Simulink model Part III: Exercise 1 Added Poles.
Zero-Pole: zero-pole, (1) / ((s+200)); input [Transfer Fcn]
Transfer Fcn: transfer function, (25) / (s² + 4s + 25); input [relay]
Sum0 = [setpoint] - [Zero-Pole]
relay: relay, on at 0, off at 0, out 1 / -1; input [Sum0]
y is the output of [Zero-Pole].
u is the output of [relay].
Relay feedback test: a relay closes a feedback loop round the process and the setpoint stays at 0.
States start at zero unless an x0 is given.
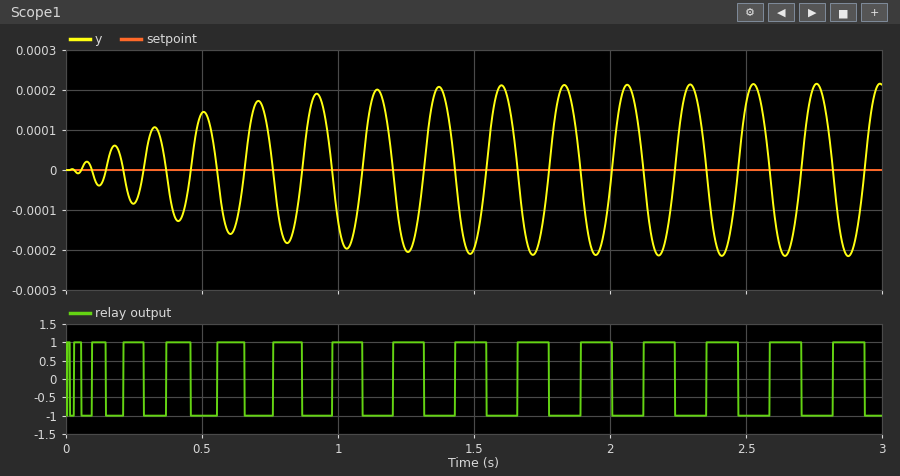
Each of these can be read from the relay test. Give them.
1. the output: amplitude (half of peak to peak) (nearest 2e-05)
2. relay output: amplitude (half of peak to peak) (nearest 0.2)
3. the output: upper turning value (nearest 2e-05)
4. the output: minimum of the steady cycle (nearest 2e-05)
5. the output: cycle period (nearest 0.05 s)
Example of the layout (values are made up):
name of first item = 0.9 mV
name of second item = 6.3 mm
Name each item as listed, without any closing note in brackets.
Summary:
the output: amplitude (half of peak to peak) = 0.00022
relay output: amplitude (half of peak to peak) = 1.0
the output: upper turning value = 0.00022
the output: minimum of the steady cycle = -0.00022
the output: cycle period = 0.25 s
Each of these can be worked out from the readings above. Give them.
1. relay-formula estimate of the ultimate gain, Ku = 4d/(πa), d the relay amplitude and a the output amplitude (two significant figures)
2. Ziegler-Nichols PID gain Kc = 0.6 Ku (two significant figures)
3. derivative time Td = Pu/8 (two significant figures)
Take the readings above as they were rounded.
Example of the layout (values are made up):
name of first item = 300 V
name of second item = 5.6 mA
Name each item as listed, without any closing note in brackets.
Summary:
relay-formula estimate of the ultimate gain, Ku = 4d/(πa), d the relay amplitude and a the output amplitude = 5800
Ziegler-Nichols PID gain Kc = 0.6 Ku = 3500
derivative time Td = Pu/8 = 0.031 s
